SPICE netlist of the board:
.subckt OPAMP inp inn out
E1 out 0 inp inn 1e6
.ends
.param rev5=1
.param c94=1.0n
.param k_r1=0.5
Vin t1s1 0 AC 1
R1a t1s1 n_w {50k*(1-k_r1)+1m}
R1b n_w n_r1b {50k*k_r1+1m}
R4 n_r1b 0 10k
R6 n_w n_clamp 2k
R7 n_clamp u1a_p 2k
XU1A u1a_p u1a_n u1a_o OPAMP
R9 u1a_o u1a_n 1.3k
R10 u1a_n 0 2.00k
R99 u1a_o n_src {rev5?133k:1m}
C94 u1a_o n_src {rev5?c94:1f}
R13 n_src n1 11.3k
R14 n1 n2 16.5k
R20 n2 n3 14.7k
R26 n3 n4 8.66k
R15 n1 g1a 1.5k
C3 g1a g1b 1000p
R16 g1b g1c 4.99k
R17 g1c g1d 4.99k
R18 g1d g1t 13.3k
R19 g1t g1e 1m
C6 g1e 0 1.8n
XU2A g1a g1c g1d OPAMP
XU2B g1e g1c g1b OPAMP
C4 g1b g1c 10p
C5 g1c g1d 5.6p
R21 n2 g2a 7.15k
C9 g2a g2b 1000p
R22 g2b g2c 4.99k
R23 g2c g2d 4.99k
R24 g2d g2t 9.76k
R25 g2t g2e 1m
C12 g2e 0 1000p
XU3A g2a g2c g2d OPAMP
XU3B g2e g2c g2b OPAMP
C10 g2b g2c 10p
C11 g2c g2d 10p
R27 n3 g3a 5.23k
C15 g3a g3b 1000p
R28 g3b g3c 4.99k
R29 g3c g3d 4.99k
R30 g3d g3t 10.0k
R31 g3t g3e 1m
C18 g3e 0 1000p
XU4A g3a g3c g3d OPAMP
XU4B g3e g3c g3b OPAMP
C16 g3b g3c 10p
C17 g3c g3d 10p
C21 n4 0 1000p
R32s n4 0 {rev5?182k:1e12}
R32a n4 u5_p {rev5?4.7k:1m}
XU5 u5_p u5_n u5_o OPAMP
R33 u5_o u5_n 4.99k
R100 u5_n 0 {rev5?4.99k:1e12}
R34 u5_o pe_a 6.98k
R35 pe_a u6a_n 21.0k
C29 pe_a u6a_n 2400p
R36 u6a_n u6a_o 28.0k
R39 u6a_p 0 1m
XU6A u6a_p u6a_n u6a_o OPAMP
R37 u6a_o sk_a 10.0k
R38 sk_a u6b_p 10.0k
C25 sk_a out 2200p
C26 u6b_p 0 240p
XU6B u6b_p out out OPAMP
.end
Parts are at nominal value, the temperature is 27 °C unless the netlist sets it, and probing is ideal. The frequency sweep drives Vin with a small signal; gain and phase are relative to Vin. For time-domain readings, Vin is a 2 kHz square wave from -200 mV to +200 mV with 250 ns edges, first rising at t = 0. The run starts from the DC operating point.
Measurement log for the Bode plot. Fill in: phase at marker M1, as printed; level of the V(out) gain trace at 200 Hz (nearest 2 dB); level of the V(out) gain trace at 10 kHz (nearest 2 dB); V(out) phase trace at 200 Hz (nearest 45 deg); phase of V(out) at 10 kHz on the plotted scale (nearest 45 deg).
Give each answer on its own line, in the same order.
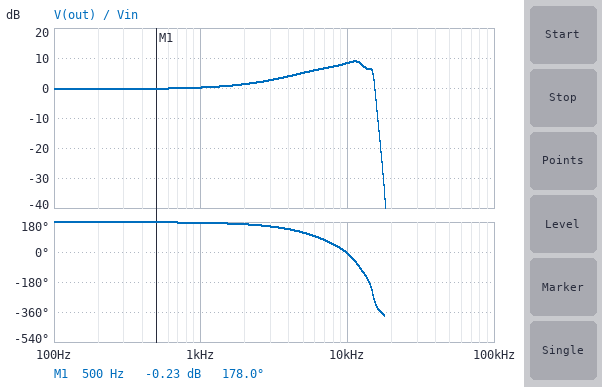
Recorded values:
178.0 deg
0 dB
8 dB
180 deg
0 deg
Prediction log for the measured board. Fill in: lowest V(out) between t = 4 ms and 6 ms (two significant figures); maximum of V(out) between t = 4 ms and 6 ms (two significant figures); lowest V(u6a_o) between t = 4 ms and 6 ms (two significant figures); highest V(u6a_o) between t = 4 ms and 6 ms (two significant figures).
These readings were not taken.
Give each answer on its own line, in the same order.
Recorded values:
-570 mV
570 mV
-520 mV
520 mV
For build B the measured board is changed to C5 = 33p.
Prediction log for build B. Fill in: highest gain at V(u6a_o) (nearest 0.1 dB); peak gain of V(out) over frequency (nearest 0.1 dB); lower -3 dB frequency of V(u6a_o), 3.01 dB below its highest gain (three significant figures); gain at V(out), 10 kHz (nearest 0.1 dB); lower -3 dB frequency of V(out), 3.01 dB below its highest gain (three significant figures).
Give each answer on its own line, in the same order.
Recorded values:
7.2 dB
9.0 dB
4.48 kHz
8.4 dB
6.07 kHz
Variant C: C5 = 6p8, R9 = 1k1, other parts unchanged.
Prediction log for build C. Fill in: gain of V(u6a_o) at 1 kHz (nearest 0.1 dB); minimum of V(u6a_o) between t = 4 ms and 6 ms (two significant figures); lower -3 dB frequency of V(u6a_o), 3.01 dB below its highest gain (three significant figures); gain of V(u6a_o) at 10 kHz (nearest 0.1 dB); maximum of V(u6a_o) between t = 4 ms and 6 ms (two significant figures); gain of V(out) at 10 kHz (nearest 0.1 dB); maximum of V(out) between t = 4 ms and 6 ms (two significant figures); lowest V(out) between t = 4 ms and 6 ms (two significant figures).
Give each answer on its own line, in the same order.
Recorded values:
-0.4 dB
-490 mV
4.39 kHz
6.3 dB
490 mV
7.8 dB
540 mV
-540 mV
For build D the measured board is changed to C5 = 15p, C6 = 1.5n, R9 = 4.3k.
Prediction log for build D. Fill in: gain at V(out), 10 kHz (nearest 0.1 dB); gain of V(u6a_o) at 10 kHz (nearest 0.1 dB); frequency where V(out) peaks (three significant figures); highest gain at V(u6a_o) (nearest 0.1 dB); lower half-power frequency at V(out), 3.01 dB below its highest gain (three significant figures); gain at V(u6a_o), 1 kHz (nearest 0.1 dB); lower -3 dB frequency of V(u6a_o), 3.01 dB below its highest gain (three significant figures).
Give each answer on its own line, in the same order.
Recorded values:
14.6 dB
13.1 dB
11.9 kHz
13.7 dB
7.28 kHz
5.7 dB
5.45 kHz
